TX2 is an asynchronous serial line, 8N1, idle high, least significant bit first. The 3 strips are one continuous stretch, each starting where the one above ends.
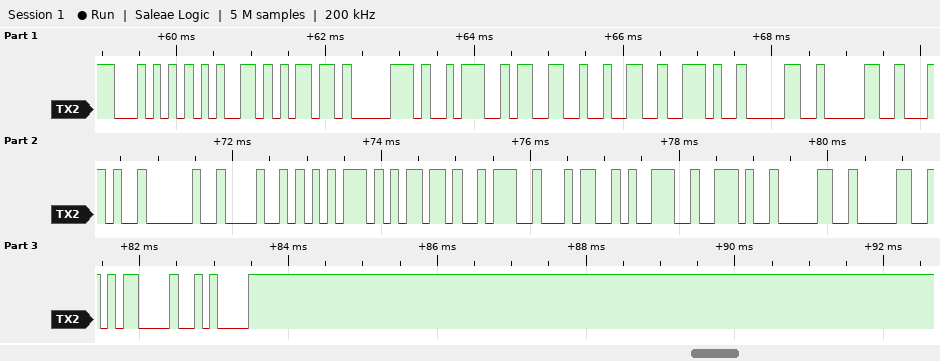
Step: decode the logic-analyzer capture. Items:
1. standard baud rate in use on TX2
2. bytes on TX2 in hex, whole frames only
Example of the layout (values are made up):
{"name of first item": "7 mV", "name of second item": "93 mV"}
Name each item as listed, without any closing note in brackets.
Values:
{"standard baud rate in use on TX2": "9600 baud", "bytes on TX2 in hex, whole frames only": "0x54 0x65 0x6D 0x70 0x3A 0x33 0x32 0x2E 0x30 0x30 0x2C 0x20 0x48 0x75 0x6D 0x3A 0x34 0x39 0x2E 0x30 0x30 0x0D 0x0A"}
